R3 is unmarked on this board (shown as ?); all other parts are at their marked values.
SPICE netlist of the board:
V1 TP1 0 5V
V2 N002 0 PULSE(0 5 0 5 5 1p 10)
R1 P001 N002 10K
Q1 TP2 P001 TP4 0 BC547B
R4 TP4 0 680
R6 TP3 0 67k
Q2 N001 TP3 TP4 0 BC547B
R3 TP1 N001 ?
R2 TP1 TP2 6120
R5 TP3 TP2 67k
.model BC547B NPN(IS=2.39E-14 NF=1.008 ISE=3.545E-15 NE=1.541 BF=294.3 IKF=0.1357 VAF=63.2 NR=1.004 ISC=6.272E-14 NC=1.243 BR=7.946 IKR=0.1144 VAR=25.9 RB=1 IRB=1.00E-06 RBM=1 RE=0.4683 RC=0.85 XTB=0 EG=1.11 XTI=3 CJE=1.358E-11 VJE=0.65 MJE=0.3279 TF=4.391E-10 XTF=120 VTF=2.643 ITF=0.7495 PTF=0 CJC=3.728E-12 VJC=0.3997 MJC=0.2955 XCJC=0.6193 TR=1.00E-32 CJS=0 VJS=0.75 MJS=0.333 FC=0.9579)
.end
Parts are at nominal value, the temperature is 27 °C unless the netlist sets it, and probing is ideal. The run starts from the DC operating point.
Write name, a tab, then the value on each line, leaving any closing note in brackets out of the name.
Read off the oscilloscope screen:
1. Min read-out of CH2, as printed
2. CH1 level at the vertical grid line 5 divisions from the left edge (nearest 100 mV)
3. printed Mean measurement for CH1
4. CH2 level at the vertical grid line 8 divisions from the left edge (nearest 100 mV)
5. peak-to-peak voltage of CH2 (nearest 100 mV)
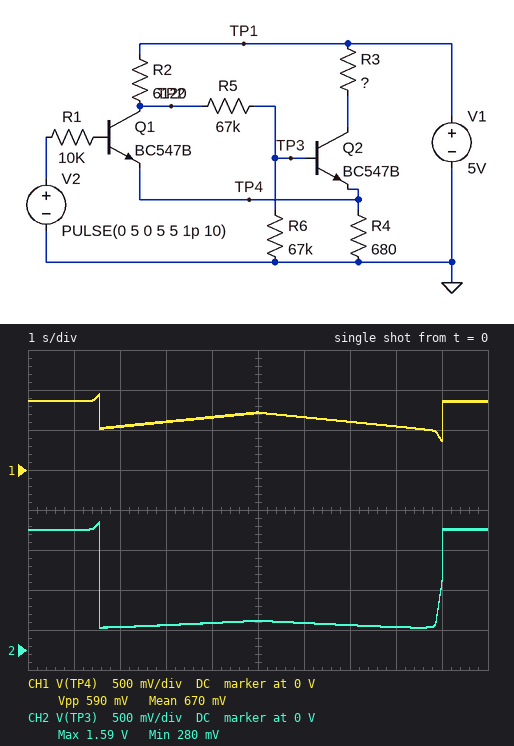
Min read-out of CH2, as printed	280 mV
CH1 level at the vertical grid line 5 divisions from the left edge	700 mV
printed Mean measurement for CH1	670 mV
CH2 level at the vertical grid line 8 divisions from the left edge	300 mV
peak-to-peak voltage of CH2	1.3 V
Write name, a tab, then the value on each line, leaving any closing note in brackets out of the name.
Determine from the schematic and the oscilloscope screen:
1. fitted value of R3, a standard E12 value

fitted value of R3, a standard E12 value	3.3 kΩ
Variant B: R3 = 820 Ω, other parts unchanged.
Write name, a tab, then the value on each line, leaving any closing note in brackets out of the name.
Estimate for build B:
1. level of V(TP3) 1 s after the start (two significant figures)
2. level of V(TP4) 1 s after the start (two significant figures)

level of V(TP3) 1 s after the start	2.1 V
level of V(TP4) 1 s after the start	1.5 V
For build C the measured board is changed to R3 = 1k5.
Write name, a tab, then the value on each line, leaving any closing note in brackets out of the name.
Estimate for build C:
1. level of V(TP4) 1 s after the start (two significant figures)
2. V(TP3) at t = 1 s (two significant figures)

level of V(TP4) 1 s after the start	1.5 V
V(TP3) at t = 1 s	2.1 V
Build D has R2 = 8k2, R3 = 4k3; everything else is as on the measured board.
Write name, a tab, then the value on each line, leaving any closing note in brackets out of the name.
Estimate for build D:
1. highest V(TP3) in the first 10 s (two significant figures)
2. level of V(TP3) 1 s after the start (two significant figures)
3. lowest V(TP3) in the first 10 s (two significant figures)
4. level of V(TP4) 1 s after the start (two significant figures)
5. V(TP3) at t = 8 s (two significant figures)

highest V(TP3) in the first 10 s	1.4 V
level of V(TP3) 1 s after the start	1.3 V
lowest V(TP3) in the first 10 s	220 mV
level of V(TP4) 1 s after the start	690 mV
V(TP3) at t = 8 s	230 mV
